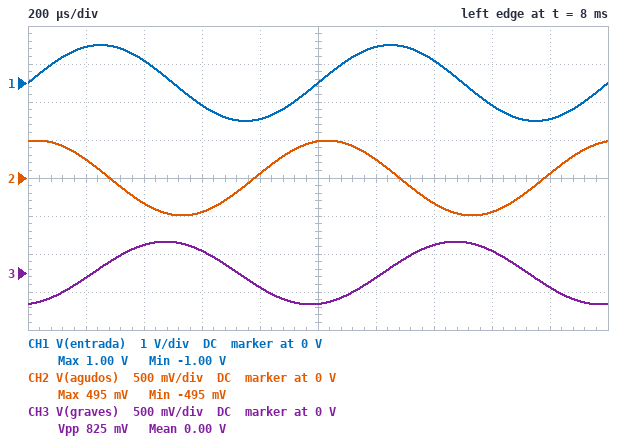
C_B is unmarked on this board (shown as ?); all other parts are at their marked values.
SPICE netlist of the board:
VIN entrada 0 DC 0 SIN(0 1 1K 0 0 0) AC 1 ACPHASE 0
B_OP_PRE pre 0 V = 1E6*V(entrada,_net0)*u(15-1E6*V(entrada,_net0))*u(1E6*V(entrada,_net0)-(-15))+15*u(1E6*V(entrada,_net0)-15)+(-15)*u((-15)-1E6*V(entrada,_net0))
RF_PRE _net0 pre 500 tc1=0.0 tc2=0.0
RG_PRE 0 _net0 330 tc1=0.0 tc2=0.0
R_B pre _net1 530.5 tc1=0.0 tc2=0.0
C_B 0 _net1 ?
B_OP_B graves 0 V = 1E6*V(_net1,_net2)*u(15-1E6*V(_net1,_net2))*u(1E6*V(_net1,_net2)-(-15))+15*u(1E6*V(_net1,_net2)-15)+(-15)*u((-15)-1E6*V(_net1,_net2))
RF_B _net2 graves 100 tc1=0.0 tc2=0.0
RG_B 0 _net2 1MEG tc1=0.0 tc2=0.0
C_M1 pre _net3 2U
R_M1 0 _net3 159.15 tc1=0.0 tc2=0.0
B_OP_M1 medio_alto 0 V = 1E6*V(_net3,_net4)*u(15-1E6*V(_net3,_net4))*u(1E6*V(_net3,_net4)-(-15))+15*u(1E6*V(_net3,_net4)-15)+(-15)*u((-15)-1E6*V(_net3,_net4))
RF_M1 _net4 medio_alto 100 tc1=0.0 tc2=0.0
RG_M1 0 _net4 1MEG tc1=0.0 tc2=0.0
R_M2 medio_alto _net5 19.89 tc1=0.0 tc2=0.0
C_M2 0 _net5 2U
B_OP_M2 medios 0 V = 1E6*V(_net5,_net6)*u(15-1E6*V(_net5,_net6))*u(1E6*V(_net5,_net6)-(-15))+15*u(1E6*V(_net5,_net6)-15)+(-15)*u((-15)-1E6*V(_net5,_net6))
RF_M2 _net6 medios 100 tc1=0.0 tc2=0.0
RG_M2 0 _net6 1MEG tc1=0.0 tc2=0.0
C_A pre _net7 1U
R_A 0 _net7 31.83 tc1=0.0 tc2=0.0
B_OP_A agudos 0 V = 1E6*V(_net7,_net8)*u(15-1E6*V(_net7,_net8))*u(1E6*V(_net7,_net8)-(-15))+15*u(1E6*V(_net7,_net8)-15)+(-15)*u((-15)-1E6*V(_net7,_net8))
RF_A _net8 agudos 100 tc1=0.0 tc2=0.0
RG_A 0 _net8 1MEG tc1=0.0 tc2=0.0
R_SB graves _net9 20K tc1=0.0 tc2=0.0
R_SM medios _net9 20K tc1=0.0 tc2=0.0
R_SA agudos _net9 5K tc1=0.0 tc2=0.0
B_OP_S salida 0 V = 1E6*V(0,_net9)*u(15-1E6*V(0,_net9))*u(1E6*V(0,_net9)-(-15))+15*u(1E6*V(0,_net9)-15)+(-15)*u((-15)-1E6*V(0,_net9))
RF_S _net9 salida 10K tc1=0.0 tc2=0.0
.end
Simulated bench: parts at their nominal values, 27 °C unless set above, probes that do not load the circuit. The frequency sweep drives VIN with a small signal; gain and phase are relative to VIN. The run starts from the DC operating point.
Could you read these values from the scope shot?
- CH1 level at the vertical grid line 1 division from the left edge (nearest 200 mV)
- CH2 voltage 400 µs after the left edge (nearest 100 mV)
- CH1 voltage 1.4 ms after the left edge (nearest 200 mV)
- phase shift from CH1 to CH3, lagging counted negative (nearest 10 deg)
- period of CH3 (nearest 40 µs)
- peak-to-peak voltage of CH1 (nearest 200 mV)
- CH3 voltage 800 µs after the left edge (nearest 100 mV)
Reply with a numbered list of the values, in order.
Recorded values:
1. 1.0 V
2. -300 mV
3. 600 mV
4. -80 deg
5. 1.00 ms
6. 2.0 V
7. -200 mV
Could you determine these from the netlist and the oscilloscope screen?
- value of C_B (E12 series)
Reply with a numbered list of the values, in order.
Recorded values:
1. 1.8 µF
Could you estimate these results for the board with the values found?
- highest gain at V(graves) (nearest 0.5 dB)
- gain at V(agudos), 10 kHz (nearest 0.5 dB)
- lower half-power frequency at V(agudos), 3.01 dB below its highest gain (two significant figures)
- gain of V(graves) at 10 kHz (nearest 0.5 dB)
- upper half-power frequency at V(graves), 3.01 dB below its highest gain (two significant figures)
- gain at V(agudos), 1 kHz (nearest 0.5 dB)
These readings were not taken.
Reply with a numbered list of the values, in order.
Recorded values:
1. 8.0 dB
2. 7.0 dB
3. 5.0 kHz
4. -27.5 dB
5. 170 Hz
6. -6.0 dB
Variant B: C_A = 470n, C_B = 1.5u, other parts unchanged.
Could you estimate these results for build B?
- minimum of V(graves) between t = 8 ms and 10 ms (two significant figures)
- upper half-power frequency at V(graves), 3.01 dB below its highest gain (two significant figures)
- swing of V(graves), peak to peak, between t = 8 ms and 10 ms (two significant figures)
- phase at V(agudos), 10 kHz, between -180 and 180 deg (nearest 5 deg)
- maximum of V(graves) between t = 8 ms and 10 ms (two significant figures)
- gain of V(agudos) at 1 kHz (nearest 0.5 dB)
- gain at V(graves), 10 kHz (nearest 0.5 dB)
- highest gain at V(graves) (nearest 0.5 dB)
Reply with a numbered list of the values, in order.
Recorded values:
1. -490 mV
2. 200 Hz
3. 990 mV
4. 45 deg
5. 490 mV
6. -12.5 dB
7. -26.0 dB
8. 8.0 dB
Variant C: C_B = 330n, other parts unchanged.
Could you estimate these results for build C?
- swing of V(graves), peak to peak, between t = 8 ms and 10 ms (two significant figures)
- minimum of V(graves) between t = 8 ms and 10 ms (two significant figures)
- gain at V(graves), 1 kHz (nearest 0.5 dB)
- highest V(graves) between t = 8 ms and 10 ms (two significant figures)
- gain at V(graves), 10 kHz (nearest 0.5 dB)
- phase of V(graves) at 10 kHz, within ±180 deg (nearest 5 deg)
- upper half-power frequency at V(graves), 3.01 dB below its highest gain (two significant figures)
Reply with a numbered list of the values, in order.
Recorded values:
1. 3.4 V
2. -1.7 V
3. 4.5 dB
4. 1.7 V
5. -13.0 dB
6. -85 deg
7. 910 Hz
